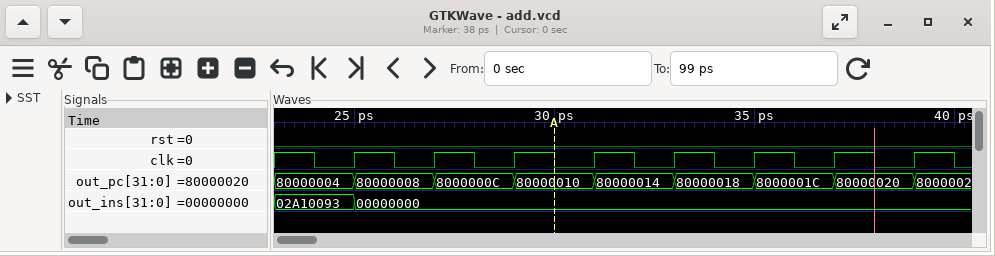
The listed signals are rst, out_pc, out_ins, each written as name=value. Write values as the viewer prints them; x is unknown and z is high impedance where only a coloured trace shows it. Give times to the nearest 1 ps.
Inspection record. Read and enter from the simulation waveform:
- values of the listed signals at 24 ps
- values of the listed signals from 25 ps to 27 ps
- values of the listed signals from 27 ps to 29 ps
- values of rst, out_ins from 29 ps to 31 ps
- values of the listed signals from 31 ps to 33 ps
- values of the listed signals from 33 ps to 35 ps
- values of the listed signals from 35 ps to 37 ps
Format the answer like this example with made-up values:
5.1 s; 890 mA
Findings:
rst=0, out_pc=80000004, out_ins=02A10093; rst=0, out_pc=80000008, out_ins=00000000; rst=0, out_pc=8000000C, out_ins=00000000; rst=0, out_ins=00000000; rst=0, out_pc=80000014, out_ins=00000000; rst=0, out_pc=80000018, out_ins=00000000; rst=0, out_pc=8000001C, out_ins=00000000
